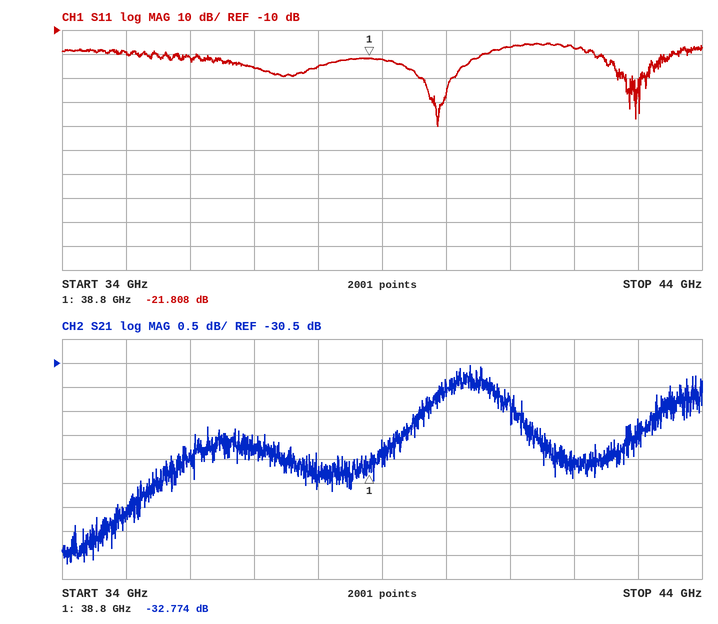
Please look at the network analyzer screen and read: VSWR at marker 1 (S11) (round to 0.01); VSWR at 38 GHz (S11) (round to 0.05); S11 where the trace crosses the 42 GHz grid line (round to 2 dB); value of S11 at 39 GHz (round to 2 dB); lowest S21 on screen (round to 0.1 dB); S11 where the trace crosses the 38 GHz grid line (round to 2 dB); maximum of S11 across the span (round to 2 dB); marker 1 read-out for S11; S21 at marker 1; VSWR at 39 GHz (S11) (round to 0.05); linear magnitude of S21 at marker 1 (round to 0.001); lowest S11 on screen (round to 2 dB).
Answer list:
1.18
1.10
-18 dB
-22 dB
-34.7 dB
-26 dB
-16 dB
-21.808 dB
-32.774 dB
1.15
0.023
-50 dB
